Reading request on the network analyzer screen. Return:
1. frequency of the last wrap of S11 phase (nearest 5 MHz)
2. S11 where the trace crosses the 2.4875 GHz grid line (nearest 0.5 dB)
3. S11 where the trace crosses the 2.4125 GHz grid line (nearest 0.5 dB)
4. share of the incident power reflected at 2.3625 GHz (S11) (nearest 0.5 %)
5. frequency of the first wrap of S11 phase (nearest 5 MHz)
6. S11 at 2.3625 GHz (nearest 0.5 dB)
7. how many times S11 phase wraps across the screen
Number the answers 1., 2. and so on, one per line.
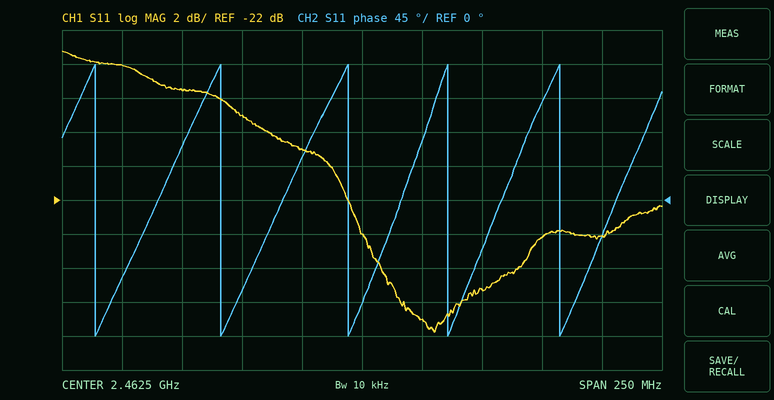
1. 2.545 GHz
2. -29.0 dB
3. -17.0 dB
4. 4.0 %
5. 2.350 GHz
6. -14.0 dB
7. 5
